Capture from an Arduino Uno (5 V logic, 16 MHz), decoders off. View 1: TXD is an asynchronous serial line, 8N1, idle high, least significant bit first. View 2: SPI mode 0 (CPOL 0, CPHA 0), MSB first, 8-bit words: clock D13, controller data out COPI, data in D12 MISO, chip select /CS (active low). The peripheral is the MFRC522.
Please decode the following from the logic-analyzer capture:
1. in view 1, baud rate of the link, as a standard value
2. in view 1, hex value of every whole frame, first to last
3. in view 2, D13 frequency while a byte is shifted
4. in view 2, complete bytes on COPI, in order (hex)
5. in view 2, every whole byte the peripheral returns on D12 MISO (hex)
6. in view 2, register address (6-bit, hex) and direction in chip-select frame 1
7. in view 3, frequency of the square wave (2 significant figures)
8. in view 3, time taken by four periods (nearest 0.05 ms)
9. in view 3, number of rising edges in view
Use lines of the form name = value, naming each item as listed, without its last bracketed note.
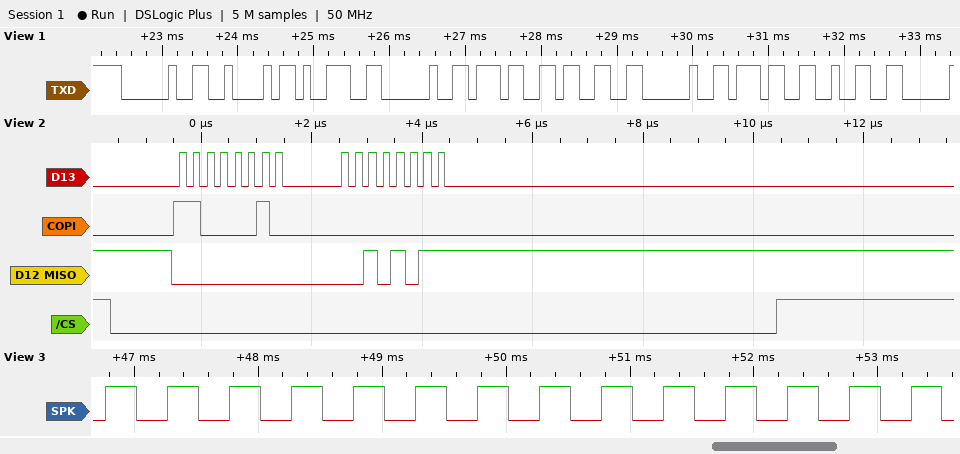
in view 1, baud rate of the link, as a standard value = 9600 baud
in view 1, hex value of every whole frame, first to last = 0x20 0x42 0x39 0x20 0x37 0x33 0x20 0x37 0x32
in view 2, D13 frequency while a byte is shifted = 4 MHz
in view 2, complete bytes on COPI, in order = 0xC2 0x00
in view 2, every whole byte the peripheral returns on D12 MISO = 0x00 0x2B
in view 2, register address (6-bit, hex) and direction in chip-select frame 1 = 0x21 read
in view 3, frequency of the square wave = 2.0 kHz
in view 3, time taken by four periods = 2.00 ms
in view 3, number of rising edges in view = 14
